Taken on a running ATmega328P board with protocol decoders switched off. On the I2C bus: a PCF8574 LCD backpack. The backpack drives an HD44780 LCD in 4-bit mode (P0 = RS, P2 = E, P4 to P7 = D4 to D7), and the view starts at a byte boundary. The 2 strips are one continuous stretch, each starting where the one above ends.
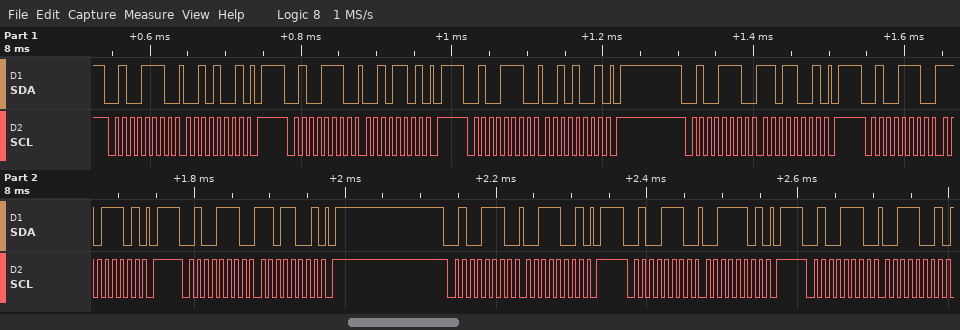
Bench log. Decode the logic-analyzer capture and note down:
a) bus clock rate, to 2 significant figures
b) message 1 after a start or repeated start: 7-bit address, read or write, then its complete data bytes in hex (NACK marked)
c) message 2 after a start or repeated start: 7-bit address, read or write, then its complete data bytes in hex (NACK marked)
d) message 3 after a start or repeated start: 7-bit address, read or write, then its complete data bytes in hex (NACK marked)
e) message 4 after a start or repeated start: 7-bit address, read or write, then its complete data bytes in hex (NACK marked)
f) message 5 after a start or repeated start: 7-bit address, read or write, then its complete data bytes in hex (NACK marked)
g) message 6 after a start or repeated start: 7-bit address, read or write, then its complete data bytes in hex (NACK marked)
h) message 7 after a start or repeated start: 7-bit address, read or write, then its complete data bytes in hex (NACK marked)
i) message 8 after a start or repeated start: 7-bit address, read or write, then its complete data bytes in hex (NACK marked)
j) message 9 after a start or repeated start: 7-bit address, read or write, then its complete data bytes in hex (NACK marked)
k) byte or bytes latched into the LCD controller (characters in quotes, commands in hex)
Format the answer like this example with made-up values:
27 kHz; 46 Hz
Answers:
100 kHz; 0x27 write: 29; 0x27 write: 2D; 0x27 write: 29; 0x27 write: D9; 0x27 write: DD; 0x27 write: D9; 0x27 write: 39; 0x27 write: 3D; 0x27 write: 39; '-'
